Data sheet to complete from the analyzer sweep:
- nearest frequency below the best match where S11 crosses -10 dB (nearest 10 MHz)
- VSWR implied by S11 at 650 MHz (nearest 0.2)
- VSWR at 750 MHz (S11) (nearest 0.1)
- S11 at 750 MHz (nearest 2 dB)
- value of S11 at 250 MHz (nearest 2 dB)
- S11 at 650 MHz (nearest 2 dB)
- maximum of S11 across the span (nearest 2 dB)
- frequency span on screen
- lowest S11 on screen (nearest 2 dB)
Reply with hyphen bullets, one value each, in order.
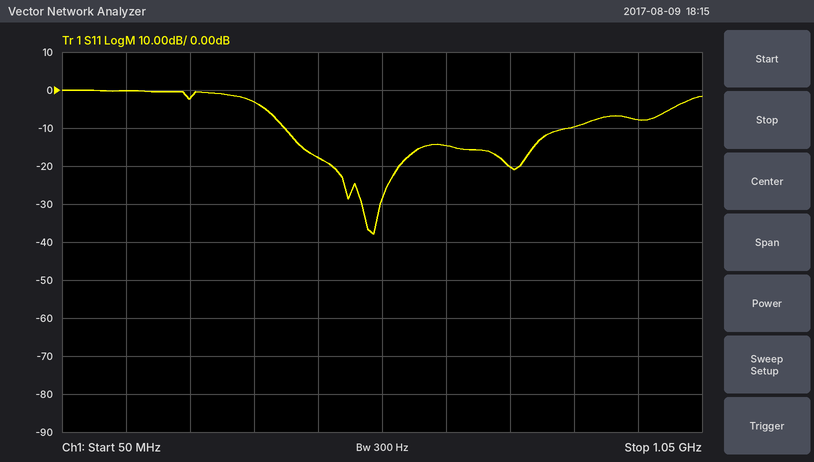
- 400 MHz
- 1.4
- 1.2
- -20 dB
- -2 dB
- -14 dB
- 0 dB
- 1 GHz
- -38 dB
